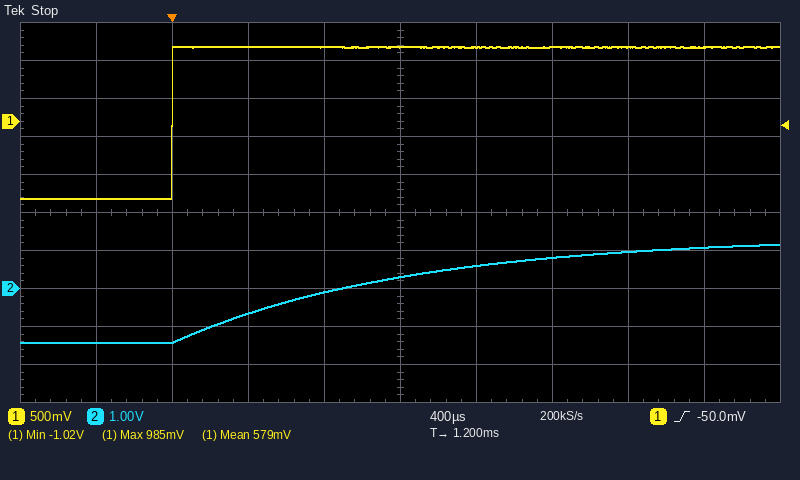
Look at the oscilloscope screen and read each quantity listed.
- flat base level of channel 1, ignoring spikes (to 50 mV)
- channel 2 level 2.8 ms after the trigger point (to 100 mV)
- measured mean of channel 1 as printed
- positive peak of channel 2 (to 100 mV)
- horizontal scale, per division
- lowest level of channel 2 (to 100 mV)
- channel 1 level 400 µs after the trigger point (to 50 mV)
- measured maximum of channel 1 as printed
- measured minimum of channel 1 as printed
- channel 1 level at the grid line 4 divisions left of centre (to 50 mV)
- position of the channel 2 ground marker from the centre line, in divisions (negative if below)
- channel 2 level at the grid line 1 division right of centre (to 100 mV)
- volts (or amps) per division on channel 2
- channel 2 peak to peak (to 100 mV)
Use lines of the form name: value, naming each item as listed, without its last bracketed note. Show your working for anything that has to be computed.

flat base level of channel 1, ignoring spikes: -1.00 V
channel 2 level 2.8 ms after the trigger point: 1.1 V
measured mean of channel 1 as printed: 579 mV
positive peak of channel 2: 1.2 V
horizontal scale, per division: 400 µs
lowest level of channel 2: -1.4 V
channel 1 level 400 µs after the trigger point: 1.00 V
measured maximum of channel 1 as printed: 985 mV
measured minimum of channel 1 as printed: -1.02 V
channel 1 level at the grid line 4 divisions left of centre: -1.00 V
position of the channel 2 ground marker from the centre line, in divisions: -2.0 div
channel 2 level at the grid line 1 division right of centre: 600 mV
volts (or amps) per division on channel 2: 1 V
channel 2 peak to peak: 1.2 V − (-1.4 V) = 2.6 V
